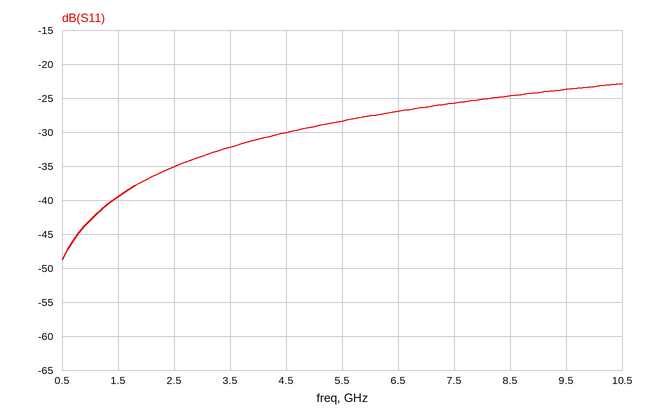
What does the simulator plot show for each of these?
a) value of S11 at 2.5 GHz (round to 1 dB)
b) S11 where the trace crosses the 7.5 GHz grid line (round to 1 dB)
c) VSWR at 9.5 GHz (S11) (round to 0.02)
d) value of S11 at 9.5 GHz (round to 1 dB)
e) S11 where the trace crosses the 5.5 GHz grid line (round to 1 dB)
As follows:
-35 dB
-26 dB
1.14
-24 dB
-28 dB
